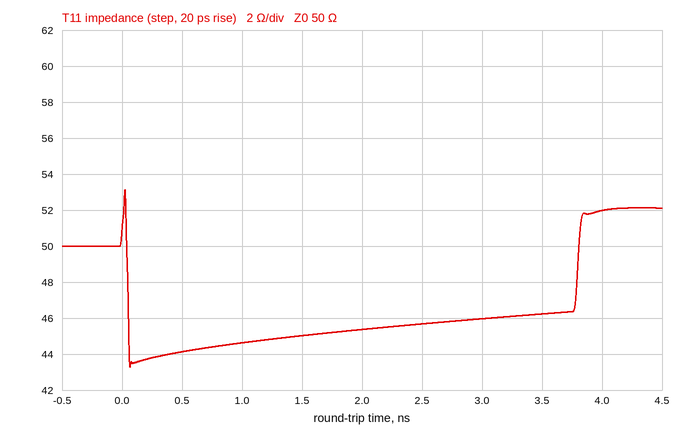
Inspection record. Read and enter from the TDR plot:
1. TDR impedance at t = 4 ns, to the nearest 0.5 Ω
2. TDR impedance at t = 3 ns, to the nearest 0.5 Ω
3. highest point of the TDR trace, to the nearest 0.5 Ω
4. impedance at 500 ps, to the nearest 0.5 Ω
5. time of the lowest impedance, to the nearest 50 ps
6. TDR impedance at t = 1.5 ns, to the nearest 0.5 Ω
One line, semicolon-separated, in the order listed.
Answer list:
52.0 Ω; 46.0 Ω; 53.0 Ω; 44.0 Ω; 50 ps; 45.0 Ω
